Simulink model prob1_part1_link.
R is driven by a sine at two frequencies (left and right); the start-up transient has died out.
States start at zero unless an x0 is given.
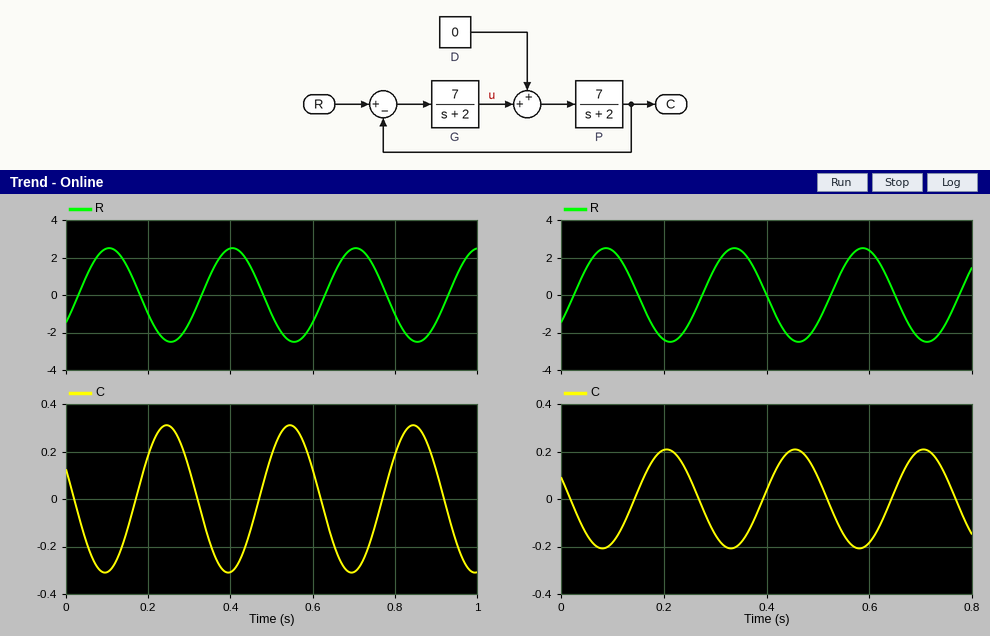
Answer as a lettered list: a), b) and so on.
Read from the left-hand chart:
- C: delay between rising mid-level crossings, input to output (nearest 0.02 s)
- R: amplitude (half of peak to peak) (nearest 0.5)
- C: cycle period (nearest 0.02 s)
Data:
a) 0.14 s
b) 2.5
c) 0.30 s
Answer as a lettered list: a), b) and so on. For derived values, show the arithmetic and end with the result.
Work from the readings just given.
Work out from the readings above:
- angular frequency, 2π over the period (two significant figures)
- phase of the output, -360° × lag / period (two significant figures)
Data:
a) 2π / 0.3 = 21 rad/s
b) -360 × 0.14 / 0.3 = -170°
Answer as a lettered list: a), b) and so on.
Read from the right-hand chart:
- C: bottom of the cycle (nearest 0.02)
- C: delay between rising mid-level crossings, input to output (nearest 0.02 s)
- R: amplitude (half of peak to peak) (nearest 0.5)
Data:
a) -0.20
b) 0.12 s
c) 2.5
